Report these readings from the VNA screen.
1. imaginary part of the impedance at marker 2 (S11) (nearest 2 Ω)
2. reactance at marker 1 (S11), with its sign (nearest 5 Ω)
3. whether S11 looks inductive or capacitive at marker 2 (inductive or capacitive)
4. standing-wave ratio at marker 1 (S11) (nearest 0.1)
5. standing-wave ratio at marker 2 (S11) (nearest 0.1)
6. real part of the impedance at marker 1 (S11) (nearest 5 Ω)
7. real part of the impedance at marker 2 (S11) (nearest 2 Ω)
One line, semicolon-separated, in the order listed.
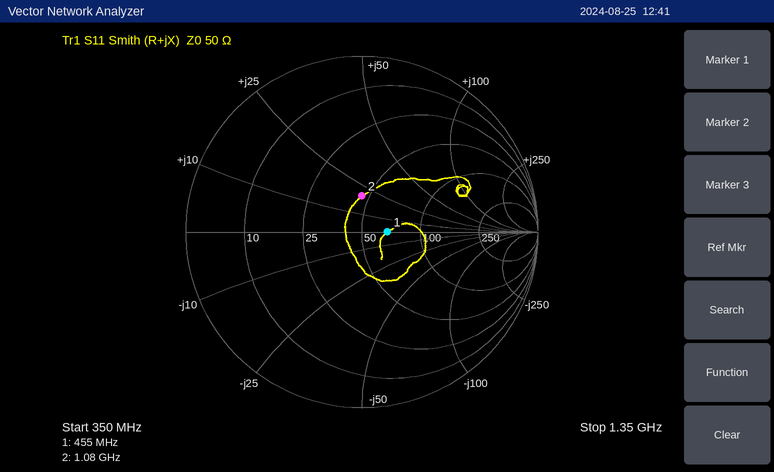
+20 Ω; 0 Ω; inductive; 1.3; 1.5; 65 Ω; 46 Ω
